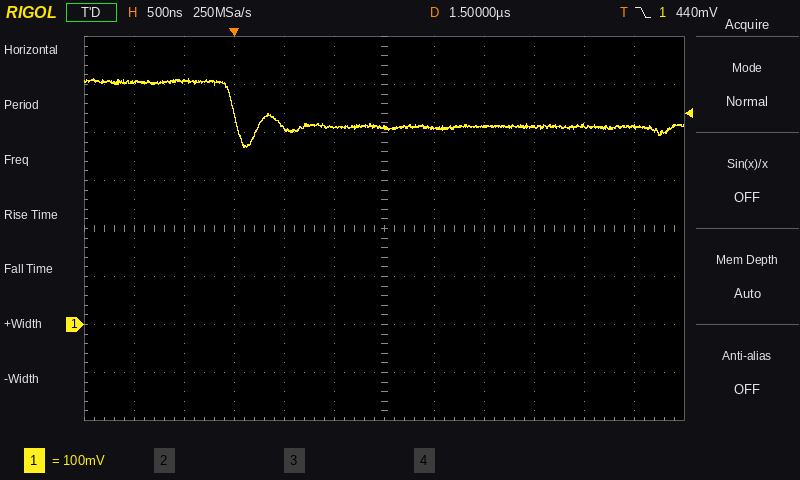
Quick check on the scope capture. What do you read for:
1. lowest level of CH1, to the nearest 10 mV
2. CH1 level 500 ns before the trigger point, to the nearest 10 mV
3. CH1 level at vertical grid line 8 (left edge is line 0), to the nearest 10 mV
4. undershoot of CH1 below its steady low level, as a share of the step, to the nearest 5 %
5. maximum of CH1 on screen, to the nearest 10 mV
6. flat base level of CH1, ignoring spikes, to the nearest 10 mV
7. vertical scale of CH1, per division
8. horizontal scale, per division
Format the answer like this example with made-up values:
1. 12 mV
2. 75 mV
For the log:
1. 370 mV
2. 510 mV
3. 410 mV
4. 45 %
5. 510 mV
6. 410 mV
7. 100 mV
8. 500 ns
